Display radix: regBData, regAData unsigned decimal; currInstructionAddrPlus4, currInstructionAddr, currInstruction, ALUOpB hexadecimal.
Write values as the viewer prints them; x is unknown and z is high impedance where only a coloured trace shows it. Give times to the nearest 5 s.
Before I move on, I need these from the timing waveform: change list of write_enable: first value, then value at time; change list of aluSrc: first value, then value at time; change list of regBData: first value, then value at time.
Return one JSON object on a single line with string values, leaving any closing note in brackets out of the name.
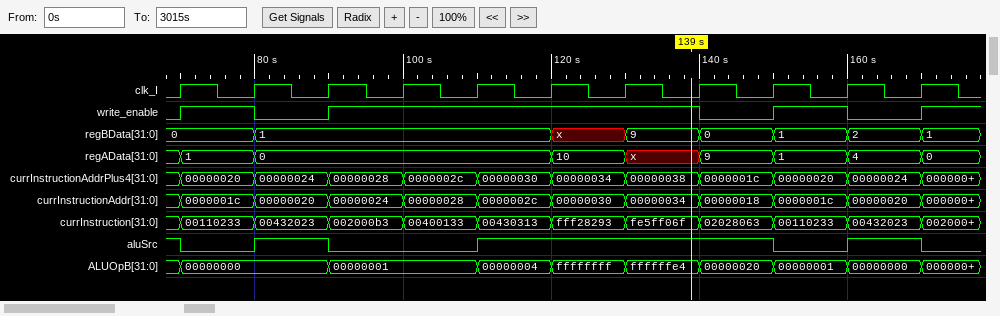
{"change list of write_enable: first value, then value at time": "0, 1 at 70 s, 0 at 80 s, 1 at 90 s, 0 at 140 s, 1 at 150 s, 0 at 160 s, 1 at 170 s", "change list of aluSrc: first value, then value at time": "1, 0 at 70 s, 1 at 80 s, 0 at 90 s, 1 at 110 s, 0 at 150 s, 1 at 160 s, 0 at 170 s", "change list of regBData: first value, then value at time": "0, 1 at 80 s, x at 120 s, 9 at 130 s, 0 at 140 s, 1 at 150 s, 2 at 160 s, 1 at 170 s"}
